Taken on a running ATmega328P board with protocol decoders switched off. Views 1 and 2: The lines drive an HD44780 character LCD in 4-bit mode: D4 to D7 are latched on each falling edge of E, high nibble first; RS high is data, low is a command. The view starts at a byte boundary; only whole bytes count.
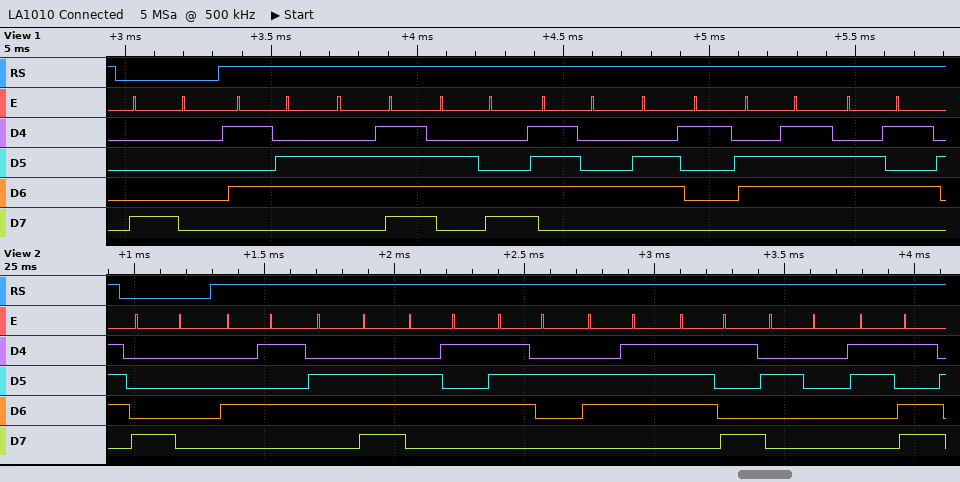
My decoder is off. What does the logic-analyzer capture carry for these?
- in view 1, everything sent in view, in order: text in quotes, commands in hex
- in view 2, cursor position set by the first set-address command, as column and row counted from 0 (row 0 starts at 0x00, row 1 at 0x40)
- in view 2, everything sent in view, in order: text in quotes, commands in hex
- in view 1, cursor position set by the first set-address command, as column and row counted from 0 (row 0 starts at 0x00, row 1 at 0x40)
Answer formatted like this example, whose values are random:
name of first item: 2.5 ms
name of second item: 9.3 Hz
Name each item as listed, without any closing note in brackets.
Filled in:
in view 1, everything sent in view, in order: text in quotes, commands in hex: 0x80 "Voltage"
in view 2, cursor position set by the first set-address command, as column and row counted from 0: column 0, row 0
in view 2, everything sent in view, in order: text in quotes, commands in hex: 0x80 "Energy ="
in view 1, cursor position set by the first set-address command, as column and row counted from 0: column 0, row 0
